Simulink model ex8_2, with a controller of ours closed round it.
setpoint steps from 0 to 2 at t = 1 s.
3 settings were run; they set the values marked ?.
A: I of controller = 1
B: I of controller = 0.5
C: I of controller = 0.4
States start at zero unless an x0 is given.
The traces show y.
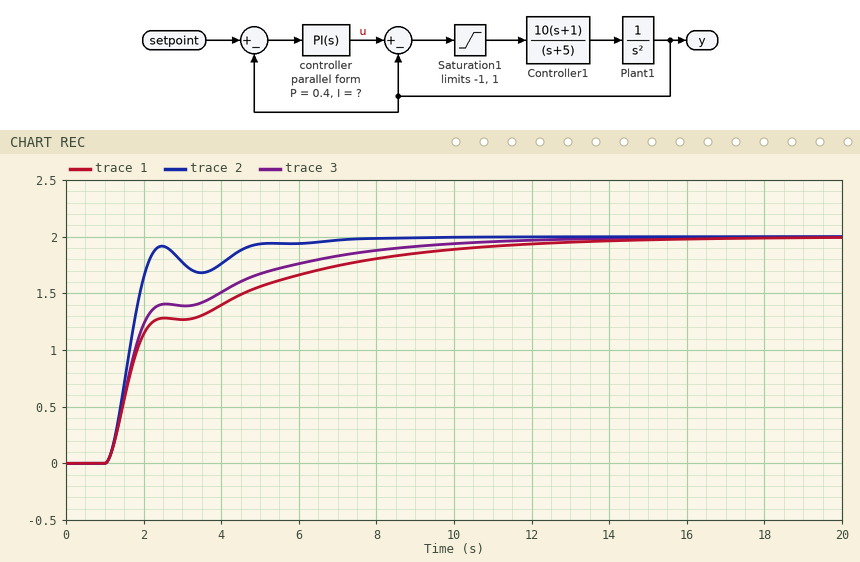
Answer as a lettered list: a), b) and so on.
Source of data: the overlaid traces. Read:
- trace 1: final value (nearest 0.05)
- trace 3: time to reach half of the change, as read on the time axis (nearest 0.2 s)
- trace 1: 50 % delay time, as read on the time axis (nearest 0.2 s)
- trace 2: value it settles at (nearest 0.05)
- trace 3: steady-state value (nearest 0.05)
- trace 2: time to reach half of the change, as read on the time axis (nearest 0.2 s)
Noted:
a) 2.00
b) 1.8 s
c) 1.8 s
d) 2.00
e) 2.00
f) 1.6 s
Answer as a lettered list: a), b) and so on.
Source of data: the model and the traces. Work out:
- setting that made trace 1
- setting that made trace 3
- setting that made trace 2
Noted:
a) C
b) B
c) A
